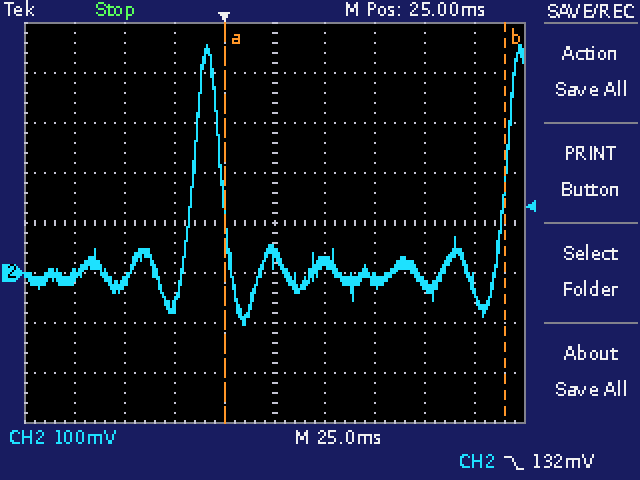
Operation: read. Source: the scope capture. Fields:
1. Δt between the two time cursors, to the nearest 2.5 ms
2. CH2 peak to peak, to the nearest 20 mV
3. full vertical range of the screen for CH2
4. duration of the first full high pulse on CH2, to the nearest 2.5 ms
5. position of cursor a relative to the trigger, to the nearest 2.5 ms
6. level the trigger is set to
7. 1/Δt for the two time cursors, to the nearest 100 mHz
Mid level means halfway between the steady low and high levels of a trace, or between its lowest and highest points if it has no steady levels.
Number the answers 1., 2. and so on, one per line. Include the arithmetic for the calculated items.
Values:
1. 140.0 ms
2. 560 mV
3. 800 mV
4. 15.0 ms
5. 0.0 ms
6. 132 mV
7. 1 / 140.0 ms ≈ 7.1 Hz
